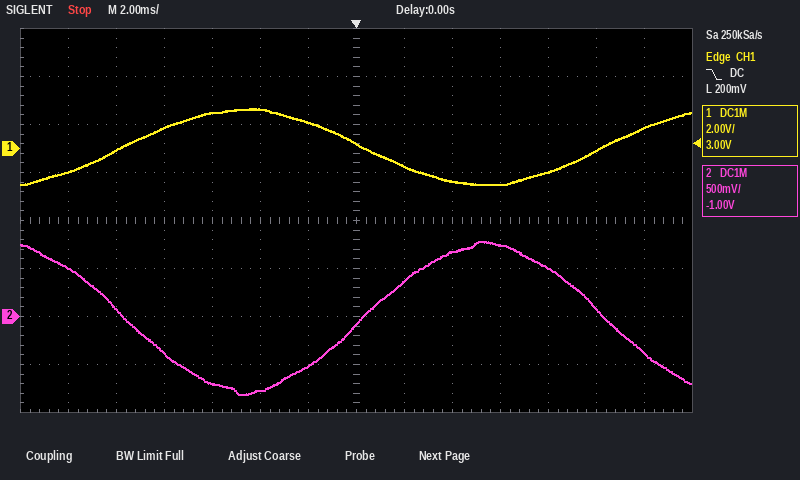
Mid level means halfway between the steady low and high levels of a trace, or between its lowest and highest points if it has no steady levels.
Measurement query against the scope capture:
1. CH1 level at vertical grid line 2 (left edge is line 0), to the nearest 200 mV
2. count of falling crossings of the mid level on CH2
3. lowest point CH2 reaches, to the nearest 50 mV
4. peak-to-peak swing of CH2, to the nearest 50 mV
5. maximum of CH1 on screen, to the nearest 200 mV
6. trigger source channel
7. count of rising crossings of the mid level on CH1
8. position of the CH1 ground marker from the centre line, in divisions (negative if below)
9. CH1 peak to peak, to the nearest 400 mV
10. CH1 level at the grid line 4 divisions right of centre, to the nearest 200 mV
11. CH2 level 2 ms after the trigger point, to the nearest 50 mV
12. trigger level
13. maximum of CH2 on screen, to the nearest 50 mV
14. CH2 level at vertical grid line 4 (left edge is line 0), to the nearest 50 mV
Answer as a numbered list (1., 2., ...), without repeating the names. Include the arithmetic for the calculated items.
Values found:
1. 0.0 V
2. 2
3. -800 mV
4. 800 mV − (-800 mV) = 1.60 V
5. 1.6 V
6. CH1
7. 2
8. +1.5 div
9. 3.2 V
10. -1.0 V
11. 350 mV
12. 200 mV
13. 800 mV
14. -700 mV
